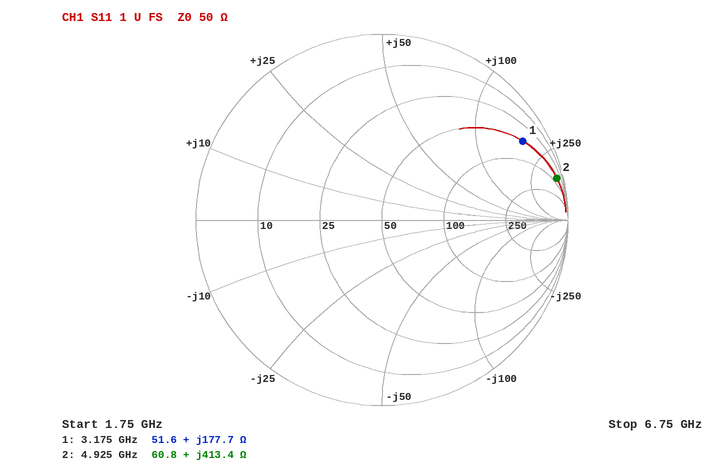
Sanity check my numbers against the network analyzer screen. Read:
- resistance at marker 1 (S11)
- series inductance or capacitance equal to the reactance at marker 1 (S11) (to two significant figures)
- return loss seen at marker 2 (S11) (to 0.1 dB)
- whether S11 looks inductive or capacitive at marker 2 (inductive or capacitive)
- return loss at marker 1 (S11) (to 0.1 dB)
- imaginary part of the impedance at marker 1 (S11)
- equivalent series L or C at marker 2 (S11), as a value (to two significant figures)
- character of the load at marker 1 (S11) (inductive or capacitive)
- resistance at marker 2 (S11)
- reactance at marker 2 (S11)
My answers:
51.6 Ω
8.9 nH
0.3 dB
inductive
1.2 dB
+177.7 Ω
13 nH
inductive
60.8 Ω
+413.4 Ω
